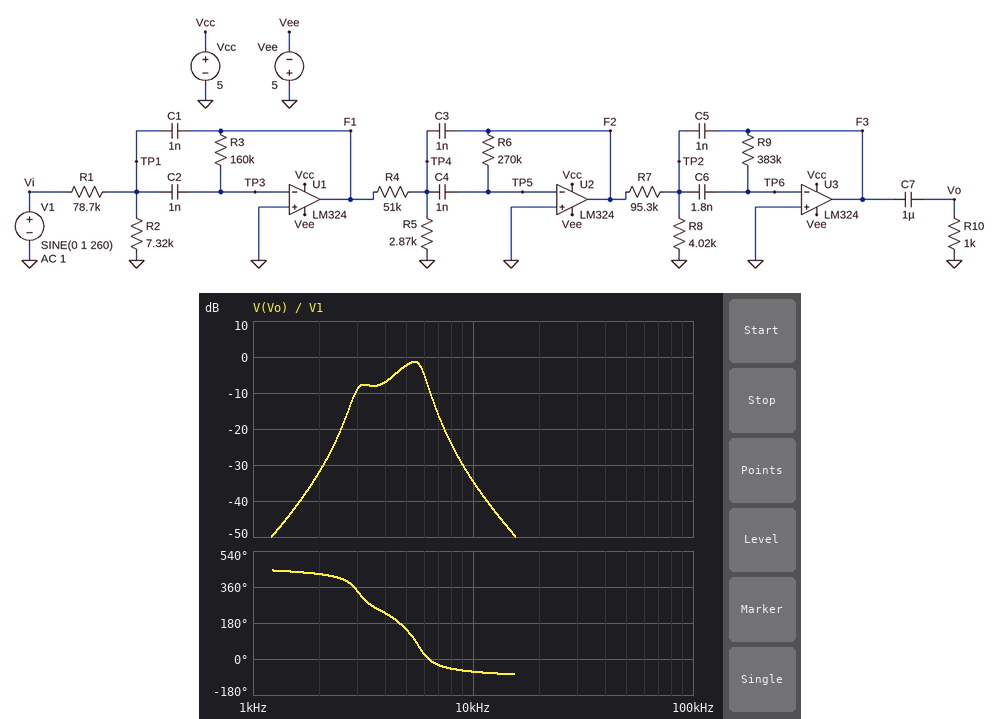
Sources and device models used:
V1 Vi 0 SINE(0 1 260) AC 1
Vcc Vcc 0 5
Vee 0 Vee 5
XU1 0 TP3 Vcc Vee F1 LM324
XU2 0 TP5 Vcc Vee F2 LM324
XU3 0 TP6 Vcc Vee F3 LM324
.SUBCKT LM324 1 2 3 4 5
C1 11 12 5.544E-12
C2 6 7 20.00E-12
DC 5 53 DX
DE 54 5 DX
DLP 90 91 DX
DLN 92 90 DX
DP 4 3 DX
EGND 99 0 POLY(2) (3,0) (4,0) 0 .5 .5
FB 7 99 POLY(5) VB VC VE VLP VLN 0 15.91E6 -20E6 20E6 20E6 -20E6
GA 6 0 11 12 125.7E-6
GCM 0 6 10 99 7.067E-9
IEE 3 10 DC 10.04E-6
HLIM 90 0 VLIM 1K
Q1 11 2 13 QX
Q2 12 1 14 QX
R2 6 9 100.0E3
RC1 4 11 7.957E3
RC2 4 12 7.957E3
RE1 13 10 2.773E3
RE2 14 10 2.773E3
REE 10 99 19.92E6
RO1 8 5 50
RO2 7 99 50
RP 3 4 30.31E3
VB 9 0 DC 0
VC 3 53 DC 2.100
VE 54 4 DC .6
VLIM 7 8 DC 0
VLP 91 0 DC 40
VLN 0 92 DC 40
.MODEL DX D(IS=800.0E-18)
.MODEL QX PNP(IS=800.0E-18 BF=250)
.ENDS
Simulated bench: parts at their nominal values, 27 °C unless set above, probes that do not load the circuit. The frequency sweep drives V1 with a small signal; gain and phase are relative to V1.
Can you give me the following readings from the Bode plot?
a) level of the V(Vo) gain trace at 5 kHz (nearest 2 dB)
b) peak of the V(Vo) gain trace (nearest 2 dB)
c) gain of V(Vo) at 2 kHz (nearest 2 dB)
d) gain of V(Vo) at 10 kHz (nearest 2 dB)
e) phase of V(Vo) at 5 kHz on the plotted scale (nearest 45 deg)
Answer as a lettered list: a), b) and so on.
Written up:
a) -2 dB
b) -2 dB
c) -32 dB
d) -34 dB
e) 135 deg
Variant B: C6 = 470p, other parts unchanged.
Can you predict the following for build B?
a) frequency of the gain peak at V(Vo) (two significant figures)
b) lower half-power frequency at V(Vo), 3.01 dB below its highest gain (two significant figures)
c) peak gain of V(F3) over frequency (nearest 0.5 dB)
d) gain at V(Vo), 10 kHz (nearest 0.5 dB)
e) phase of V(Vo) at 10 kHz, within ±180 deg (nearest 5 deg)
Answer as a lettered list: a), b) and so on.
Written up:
a) 5.7 kHz
b) 5.3 kHz
c) 8.0 dB
d) -31.5 dB
e) -55 deg
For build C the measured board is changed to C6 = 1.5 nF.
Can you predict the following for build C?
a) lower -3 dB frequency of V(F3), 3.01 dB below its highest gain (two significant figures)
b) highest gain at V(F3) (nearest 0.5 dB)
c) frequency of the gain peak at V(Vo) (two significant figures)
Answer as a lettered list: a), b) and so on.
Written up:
a) 4.4 kHz
b) -0.5 dB
c) 5.4 kHz
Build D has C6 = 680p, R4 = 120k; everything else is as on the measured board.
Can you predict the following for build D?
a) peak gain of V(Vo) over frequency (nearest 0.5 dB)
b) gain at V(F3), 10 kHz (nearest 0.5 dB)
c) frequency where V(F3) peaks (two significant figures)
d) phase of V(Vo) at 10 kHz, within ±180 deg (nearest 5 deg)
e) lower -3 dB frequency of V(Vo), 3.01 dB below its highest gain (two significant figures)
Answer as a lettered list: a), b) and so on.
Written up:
a) 1.5 dB
b) -40.5 dB
c) 5.1 kHz
d) -60 deg
e) 4.7 kHz
